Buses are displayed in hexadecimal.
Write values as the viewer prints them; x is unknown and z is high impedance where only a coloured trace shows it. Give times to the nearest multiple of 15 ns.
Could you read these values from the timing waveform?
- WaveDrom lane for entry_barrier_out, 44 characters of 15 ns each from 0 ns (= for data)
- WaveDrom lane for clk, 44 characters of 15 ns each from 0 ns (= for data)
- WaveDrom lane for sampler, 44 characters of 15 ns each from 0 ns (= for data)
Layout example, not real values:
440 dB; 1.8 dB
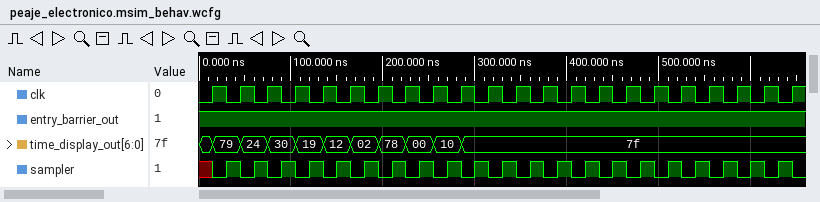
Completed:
{name: 'entry_barrier_out', wave: '1...........................................'}; {name: 'clk', wave: '01010101010101010101010101010101010101010101'}; {name: 'sampler', wave: 'x0101010101010101010101010101010101010101010'}
